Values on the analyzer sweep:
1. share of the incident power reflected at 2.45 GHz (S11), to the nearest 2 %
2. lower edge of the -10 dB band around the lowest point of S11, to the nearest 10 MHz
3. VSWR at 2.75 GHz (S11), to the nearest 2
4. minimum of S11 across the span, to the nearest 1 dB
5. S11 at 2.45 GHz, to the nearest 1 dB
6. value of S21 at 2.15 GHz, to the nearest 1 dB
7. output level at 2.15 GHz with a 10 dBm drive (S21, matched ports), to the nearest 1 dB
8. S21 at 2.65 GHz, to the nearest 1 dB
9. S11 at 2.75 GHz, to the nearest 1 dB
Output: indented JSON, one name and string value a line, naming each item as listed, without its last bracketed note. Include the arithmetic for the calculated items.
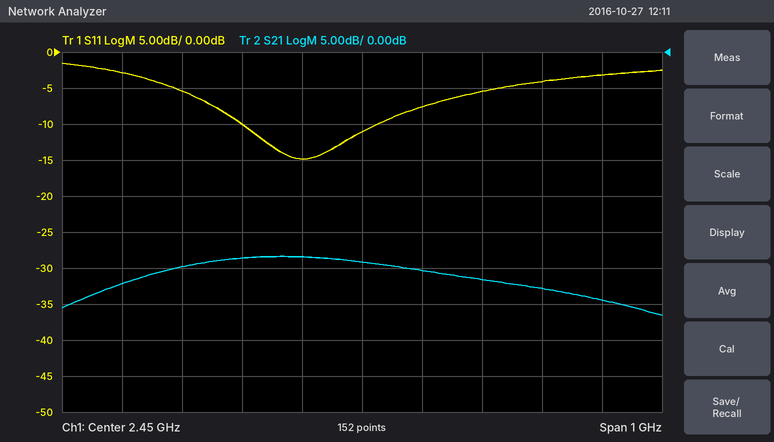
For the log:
{
  "share of the incident power reflected at 2.45 GHz (S11), to the nearest 2 %": "10^(-11/10) ≈ 8 %",
  "lower edge of the -10 dB band around the lowest point of S11, to the nearest 10 MHz": "2.25 GHz",
  "VSWR at 2.75 GHz (S11), to the nearest 2": "|Γ| = 10^(-4/20) = 0.6310; VSWR = (1 + 0.6310)/(1 − 0.6310) ≈ 4",
  "minimum of S11 across the span, to the nearest 1 dB": "-15 dB",
  "S11 at 2.45 GHz, to the nearest 1 dB": "-11 dB",
  "value of S21 at 2.15 GHz, to the nearest 1 dB": "-30 dB",
  "output level at 2.15 GHz with a 10 dBm drive (S21, matched ports), to the nearest 1 dB": "10 dBm + (-30 dB) = -20 dBm",
  "S21 at 2.65 GHz, to the nearest 1 dB": "-32 dB",
  "S11 at 2.75 GHz, to the nearest 1 dB": "-4 dB"
}
